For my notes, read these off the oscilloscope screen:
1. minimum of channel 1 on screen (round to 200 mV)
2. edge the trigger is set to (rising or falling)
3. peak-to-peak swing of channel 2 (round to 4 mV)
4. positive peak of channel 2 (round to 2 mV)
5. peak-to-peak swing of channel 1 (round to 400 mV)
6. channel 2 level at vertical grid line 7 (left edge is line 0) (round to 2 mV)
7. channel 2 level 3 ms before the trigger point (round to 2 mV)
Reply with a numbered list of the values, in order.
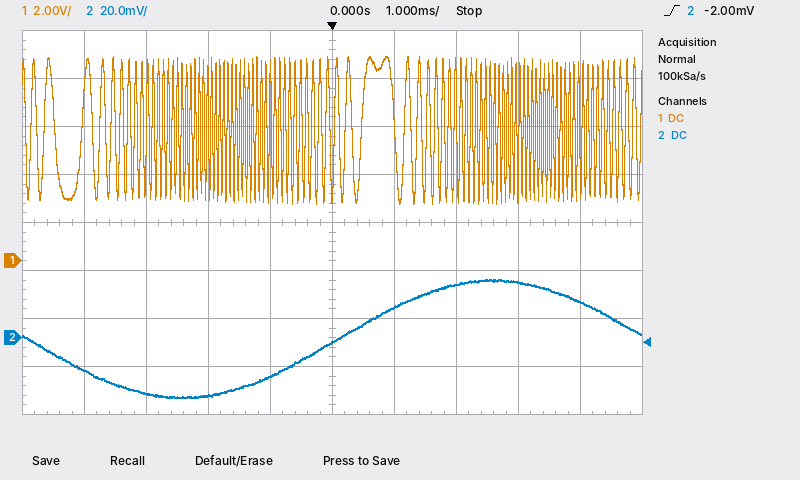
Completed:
1. 2.4 V
2. rising
3. 48 mV
4. 24 mV
5. 6.0 V
6. 22 mV
7. -24 mV
